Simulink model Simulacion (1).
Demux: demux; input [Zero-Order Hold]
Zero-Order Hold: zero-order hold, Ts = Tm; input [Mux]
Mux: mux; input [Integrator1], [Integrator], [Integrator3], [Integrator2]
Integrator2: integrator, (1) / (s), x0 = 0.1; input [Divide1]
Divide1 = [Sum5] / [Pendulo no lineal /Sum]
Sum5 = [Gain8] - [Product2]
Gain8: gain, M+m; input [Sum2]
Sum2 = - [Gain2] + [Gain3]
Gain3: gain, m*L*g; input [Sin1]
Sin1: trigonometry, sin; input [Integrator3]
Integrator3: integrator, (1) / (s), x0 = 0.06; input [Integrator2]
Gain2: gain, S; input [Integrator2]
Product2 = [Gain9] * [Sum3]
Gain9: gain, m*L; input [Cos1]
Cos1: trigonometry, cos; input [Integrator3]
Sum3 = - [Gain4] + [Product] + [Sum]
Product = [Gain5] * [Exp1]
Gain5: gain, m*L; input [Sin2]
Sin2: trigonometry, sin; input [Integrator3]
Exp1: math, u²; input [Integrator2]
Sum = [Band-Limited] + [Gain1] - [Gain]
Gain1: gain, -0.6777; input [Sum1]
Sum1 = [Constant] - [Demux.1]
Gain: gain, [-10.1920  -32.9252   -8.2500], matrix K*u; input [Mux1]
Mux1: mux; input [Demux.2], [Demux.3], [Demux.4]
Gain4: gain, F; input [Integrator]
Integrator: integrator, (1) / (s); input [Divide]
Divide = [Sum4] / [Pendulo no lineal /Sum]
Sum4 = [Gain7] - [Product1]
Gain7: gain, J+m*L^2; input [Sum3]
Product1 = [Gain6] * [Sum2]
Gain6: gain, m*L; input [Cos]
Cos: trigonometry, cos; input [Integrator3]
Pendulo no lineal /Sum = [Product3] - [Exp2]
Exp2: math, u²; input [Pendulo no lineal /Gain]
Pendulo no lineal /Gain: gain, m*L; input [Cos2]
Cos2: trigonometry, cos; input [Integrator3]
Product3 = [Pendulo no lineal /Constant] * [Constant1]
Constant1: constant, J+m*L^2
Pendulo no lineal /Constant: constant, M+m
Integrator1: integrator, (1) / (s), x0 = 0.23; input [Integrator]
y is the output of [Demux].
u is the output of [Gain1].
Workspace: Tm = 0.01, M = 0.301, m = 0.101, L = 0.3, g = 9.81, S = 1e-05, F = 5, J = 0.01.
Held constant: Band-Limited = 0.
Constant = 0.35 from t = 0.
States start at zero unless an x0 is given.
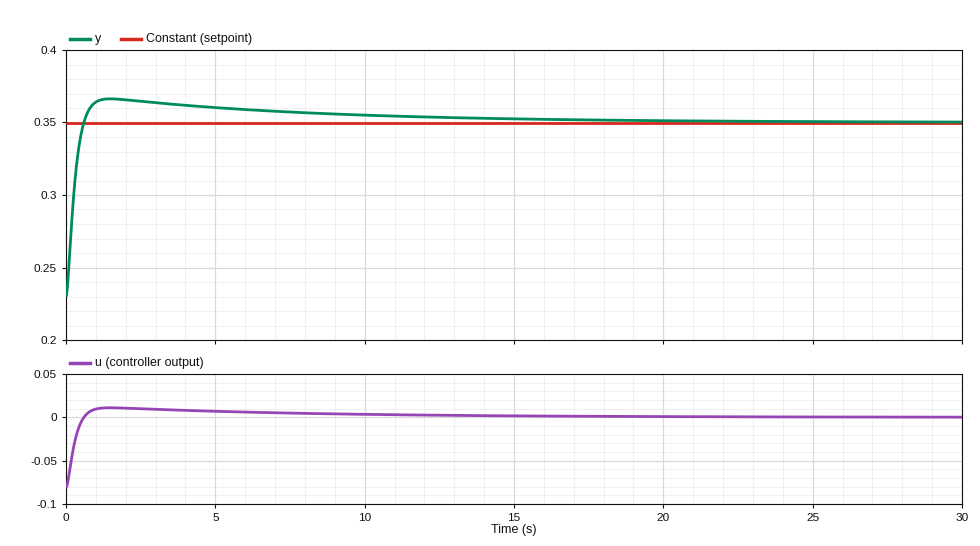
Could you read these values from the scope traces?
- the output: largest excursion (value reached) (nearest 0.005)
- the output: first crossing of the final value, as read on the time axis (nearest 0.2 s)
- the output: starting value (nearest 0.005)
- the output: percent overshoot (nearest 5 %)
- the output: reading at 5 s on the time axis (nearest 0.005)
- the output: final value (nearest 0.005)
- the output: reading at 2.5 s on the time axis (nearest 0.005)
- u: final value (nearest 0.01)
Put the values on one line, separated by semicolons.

0.365; 0.6 s; 0.230; 15 %; 0.360; 0.350; 0.365; 0.00
